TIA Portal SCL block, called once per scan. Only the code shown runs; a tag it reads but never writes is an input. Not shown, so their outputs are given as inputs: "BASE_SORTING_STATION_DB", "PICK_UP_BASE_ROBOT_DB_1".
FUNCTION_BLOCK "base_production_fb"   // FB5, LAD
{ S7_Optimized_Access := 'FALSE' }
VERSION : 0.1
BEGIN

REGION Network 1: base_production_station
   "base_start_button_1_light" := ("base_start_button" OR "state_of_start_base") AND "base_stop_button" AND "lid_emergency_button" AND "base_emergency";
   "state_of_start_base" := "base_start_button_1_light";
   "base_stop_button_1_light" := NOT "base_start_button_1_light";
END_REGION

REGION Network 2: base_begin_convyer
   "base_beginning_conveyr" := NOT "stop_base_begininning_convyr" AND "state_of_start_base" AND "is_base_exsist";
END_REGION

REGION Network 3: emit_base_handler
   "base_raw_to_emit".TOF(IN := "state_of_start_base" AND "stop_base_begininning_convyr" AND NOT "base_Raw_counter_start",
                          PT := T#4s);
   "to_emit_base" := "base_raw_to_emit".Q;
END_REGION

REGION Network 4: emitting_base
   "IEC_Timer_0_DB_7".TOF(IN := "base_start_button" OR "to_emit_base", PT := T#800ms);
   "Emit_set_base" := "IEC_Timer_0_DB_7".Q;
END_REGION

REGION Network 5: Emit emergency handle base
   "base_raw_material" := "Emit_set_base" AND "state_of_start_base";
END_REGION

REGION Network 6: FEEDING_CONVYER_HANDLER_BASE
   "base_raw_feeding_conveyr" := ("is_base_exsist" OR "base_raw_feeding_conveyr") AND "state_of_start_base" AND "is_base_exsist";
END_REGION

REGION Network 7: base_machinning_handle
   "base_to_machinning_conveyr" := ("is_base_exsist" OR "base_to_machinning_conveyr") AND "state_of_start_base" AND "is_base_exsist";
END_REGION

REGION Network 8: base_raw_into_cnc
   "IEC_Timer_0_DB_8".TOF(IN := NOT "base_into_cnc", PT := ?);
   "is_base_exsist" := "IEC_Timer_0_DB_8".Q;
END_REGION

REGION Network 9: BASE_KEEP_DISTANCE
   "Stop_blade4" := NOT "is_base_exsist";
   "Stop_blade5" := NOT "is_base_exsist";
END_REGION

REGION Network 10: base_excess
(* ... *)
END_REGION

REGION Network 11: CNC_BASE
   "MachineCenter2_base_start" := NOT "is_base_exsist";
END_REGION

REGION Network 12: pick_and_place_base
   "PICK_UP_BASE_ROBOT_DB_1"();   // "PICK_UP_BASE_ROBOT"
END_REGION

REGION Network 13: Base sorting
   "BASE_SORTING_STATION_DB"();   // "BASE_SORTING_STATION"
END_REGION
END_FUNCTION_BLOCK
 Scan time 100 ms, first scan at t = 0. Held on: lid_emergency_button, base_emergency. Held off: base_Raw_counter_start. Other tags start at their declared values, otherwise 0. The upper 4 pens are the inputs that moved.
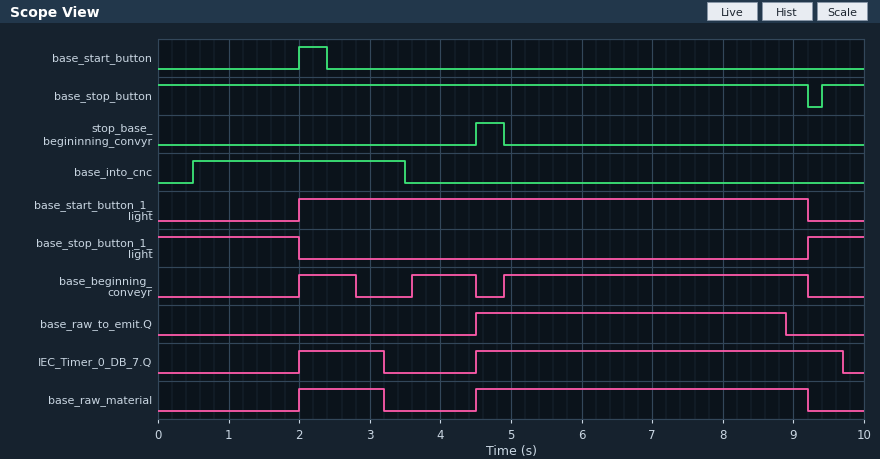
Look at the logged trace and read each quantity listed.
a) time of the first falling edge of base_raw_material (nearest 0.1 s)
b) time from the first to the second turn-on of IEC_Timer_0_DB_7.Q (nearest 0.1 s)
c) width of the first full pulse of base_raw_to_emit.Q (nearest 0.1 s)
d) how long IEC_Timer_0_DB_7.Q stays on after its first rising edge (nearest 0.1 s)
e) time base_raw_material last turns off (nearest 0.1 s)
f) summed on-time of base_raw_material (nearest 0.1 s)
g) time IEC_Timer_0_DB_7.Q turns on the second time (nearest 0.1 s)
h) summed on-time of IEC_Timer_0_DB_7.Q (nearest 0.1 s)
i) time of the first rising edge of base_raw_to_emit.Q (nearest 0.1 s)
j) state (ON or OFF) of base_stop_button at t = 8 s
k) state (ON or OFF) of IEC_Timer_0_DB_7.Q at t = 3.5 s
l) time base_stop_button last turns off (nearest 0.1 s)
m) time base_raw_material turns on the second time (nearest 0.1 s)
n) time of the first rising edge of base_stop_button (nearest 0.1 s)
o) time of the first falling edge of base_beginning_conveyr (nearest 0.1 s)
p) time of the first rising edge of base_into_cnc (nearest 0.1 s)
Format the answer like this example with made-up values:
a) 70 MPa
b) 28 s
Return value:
a) 3.2 s
b) 2.5 s
c) 4.4 s
d) 1.2 s
e) 9.2 s
f) 5.9 s
g) 4.5 s
h) 6.4 s
i) 4.5 s
j) ON
k) OFF
l) 9.2 s
m) 4.5 s
n) 9.4 s
o) 2.8 s
p) 0.5 s
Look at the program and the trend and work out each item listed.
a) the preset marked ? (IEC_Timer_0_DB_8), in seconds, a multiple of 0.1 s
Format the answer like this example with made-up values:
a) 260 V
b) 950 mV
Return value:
a) 2.2 s
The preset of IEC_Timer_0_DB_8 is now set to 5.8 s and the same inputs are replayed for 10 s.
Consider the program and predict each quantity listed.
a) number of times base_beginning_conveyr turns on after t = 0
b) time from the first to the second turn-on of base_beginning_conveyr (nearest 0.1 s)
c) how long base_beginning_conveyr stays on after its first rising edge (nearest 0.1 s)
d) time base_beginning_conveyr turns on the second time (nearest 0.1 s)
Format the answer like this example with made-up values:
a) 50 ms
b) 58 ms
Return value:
a) 2
b) 2.9 s
c) 2.5 s
d) 4.9 s
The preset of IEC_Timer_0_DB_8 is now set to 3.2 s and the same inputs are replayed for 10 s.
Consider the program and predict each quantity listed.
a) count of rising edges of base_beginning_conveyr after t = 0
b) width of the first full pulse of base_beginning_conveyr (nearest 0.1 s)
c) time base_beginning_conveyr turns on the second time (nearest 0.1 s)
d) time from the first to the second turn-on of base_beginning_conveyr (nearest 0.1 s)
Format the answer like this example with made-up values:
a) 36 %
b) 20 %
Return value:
a) 2
b) 2.5 s
c) 4.9 s
d) 2.9 s
